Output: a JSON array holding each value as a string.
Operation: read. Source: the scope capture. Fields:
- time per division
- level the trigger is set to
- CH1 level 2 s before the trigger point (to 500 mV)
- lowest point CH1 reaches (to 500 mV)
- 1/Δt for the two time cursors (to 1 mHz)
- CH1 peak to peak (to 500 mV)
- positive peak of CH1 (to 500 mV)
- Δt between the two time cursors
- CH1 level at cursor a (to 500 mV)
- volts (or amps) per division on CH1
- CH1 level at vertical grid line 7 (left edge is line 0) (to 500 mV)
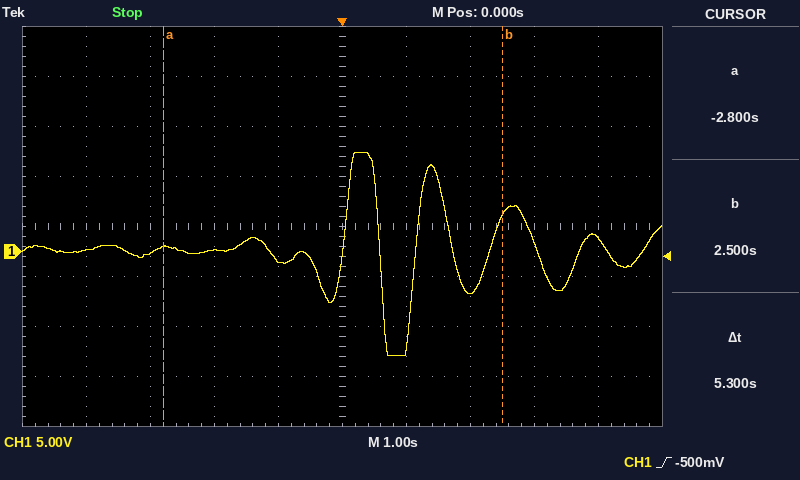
["1 s", "-500 mV", "0.0 V", "-10.5 V", "189 mHz", "20.5 V", "10.0 V", "5.3 s", "500 mV", "5 V", "-4.0 V"]
